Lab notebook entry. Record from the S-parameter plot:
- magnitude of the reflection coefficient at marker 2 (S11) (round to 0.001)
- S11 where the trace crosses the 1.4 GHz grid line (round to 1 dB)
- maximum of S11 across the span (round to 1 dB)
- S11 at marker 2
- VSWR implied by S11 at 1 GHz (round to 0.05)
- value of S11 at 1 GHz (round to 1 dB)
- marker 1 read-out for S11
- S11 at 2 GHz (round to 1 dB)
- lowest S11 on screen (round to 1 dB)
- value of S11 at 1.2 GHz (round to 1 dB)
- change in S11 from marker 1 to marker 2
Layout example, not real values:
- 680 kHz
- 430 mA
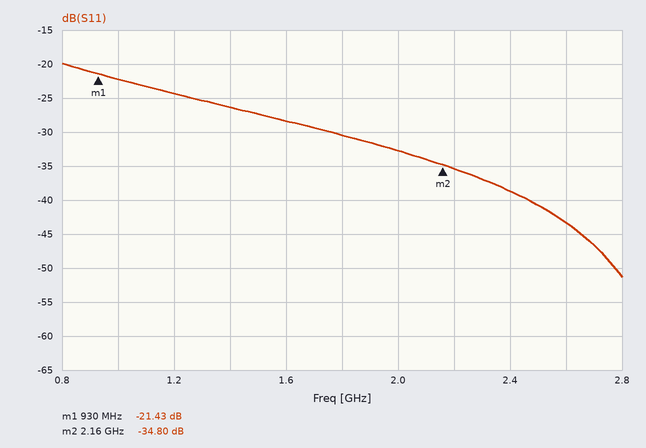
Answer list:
- 0.018
- -26 dB
- -20 dB
- -34.80 dB
- 1.15
- -22 dB
- -21.43 dB
- -33 dB
- -51 dB
- -24 dB
- -13.37 dB
